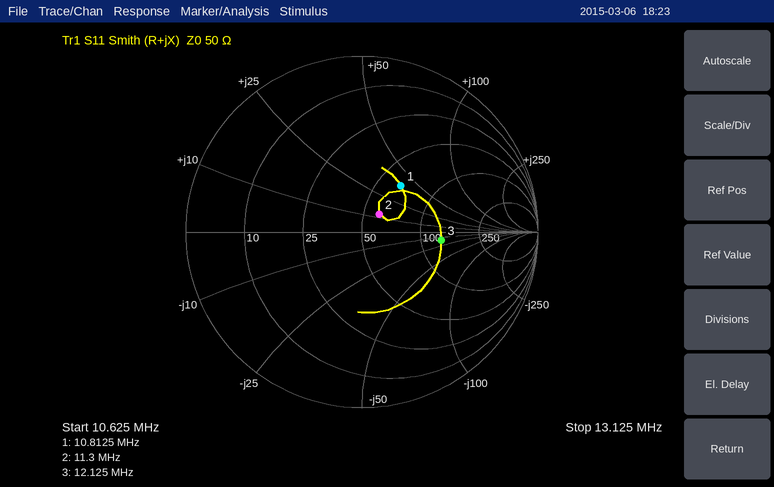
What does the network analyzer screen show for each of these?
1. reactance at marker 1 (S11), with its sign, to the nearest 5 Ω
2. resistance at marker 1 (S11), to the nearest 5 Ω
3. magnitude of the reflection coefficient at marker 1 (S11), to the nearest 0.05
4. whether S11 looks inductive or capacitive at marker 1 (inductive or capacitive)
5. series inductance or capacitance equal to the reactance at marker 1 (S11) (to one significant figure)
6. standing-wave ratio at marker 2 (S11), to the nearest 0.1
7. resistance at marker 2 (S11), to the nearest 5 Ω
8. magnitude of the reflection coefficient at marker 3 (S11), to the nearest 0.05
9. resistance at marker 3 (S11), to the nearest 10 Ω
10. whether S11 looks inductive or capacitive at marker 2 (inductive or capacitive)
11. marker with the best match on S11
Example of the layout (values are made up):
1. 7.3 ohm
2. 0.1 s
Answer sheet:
1. +40 Ω
2. 65 Ω
3. 0.35
4. inductive
5. 600 nH
6. 1.3
7. 60 Ω
8. 0.45
9. 130 Ω
10. inductive
11. marker 2
